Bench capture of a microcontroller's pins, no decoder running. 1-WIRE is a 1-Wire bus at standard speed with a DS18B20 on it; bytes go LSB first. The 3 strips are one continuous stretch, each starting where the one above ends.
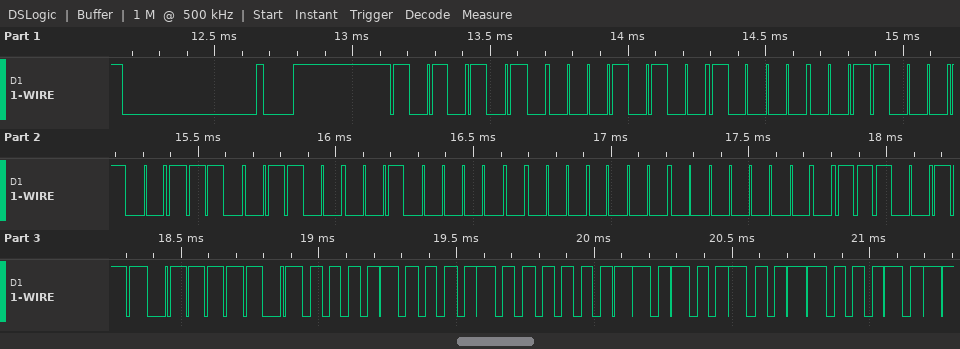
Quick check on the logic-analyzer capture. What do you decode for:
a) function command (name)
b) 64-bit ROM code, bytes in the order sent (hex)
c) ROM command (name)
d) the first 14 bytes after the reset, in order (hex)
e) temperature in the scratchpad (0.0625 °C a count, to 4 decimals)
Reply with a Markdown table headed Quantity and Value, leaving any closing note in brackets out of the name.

| Quantity | Value |
|---|---|
| function command | Read Scratchpad |
| 64-bit ROM code, bytes in the order sent | 28 81 91 33 04 00 00 E7 |
| ROM command | Match ROM |
| the first 14 bytes after the reset, in order | 55 28 81 91 33 04 00 00 E7 BE 10 02 4B 46 |
| temperature in the scratchpad | 33.0000 °C |
